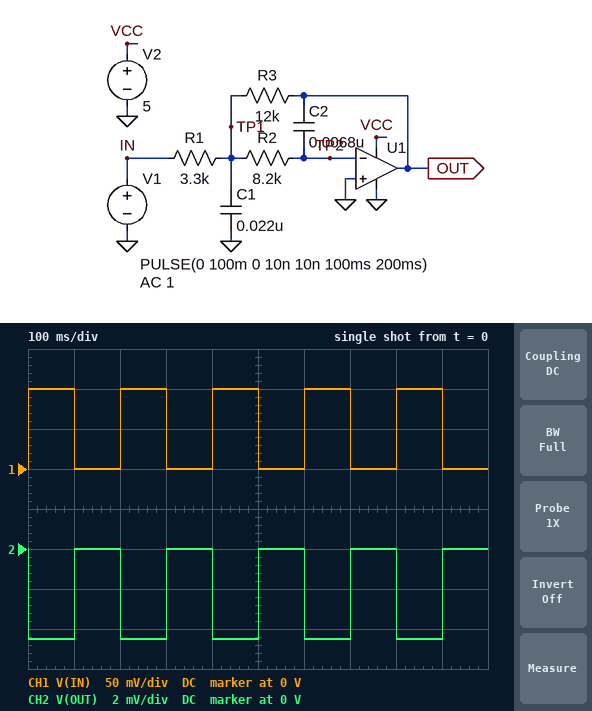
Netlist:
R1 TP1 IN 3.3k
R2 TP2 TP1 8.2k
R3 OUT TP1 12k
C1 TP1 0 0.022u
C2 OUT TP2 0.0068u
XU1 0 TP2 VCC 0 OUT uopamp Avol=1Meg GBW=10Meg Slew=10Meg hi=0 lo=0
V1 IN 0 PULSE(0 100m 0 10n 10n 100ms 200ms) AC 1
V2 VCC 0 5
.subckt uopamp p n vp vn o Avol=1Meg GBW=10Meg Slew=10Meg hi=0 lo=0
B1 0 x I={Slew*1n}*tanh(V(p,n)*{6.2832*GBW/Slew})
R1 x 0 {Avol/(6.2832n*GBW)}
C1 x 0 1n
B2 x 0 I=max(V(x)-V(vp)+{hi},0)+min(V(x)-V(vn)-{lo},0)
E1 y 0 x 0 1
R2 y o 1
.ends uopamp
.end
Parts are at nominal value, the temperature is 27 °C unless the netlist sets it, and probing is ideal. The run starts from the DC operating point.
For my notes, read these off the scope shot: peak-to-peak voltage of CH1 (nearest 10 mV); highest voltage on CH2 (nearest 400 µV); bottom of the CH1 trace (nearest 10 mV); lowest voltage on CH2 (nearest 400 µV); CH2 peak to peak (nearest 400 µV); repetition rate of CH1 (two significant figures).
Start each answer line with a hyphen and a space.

- 100 mV
- 0 V
- 0 V
- -4.4 mV
- 4.4 mV
- 5.0 Hz
